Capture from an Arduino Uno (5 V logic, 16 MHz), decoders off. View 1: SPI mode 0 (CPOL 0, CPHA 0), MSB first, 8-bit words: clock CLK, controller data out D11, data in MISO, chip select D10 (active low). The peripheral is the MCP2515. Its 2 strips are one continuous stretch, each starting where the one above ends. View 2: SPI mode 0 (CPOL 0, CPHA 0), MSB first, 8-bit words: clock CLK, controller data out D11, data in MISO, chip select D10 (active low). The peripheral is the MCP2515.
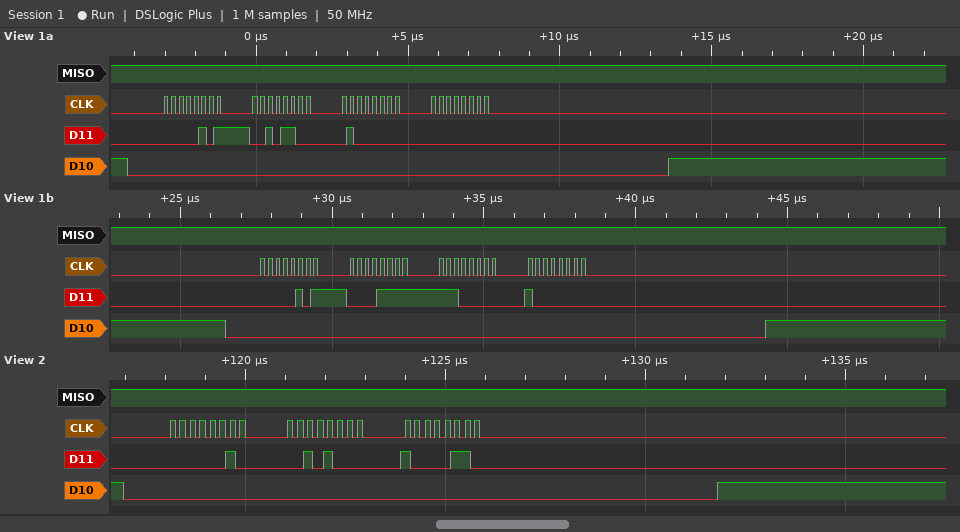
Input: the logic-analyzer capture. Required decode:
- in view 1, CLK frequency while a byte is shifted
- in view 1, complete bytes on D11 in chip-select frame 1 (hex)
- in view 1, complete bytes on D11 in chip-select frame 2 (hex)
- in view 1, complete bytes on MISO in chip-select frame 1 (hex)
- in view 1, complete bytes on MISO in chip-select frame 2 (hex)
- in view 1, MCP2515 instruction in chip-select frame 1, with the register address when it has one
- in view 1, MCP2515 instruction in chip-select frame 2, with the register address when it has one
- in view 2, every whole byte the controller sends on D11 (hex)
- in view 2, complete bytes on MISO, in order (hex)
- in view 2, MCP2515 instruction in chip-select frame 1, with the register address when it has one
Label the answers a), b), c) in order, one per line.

a) 4 MHz
b) 05 2C 40 00
c) 05 0F E0 80
d) FF FF FF FF
e) FF FF FF FF
f) BIT MODIFY 0x2C
g) BIT MODIFY 0x0F
h) 02 28 86
i) FF FF FF
j) WRITE 0x28
